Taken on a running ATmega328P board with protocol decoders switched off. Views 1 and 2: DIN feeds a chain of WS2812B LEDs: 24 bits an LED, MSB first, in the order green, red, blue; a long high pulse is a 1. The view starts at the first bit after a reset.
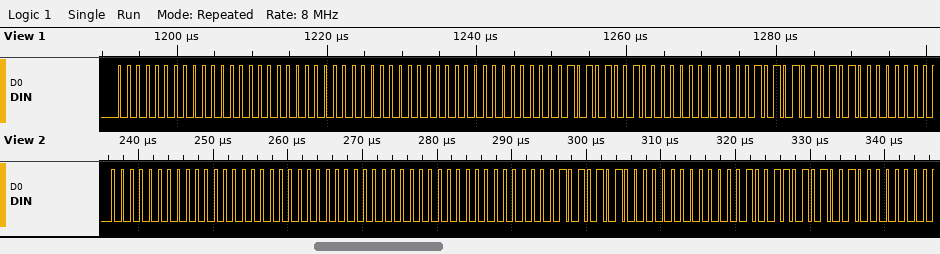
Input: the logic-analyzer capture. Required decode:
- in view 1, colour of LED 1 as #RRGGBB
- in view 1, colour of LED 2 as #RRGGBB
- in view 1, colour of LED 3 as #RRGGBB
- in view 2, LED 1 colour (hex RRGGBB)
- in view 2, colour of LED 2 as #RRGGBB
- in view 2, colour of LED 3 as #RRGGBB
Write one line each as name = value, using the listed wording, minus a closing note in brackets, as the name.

in view 1, colour of LED 1 as #RRGGBB = #000000
in view 1, colour of LED 2 as #RRGGBB = #000000
in view 1, colour of LED 3 as #RRGGBB = #00A90A
in view 2, LED 1 colour = #000000
in view 2, colour of LED 2 as #RRGGBB = #000000
in view 2, colour of LED 3 as #RRGGBB = #00AA09
